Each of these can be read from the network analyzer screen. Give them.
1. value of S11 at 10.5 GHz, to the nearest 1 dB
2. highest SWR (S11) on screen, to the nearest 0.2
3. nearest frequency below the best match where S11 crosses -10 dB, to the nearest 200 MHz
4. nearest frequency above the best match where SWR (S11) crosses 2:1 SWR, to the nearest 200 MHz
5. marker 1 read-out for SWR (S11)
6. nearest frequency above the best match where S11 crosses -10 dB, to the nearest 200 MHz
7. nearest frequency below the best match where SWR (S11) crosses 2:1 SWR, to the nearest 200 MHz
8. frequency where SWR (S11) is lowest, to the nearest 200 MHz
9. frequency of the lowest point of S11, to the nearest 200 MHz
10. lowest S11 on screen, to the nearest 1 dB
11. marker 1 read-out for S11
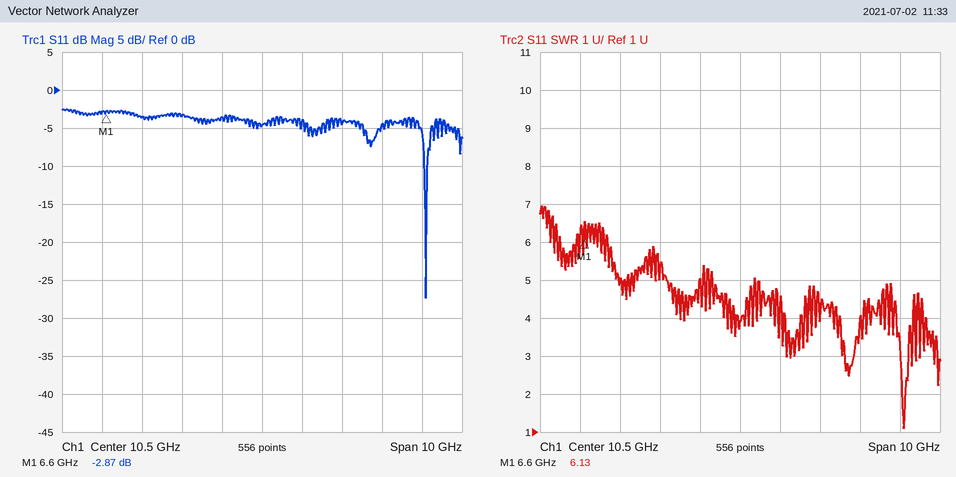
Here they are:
-5 dB
7.0
14.6 GHz
14.6 GHz
6.13
14.6 GHz
14.6 GHz
14.6 GHz
14.6 GHz
-27 dB
-2.87 dB
